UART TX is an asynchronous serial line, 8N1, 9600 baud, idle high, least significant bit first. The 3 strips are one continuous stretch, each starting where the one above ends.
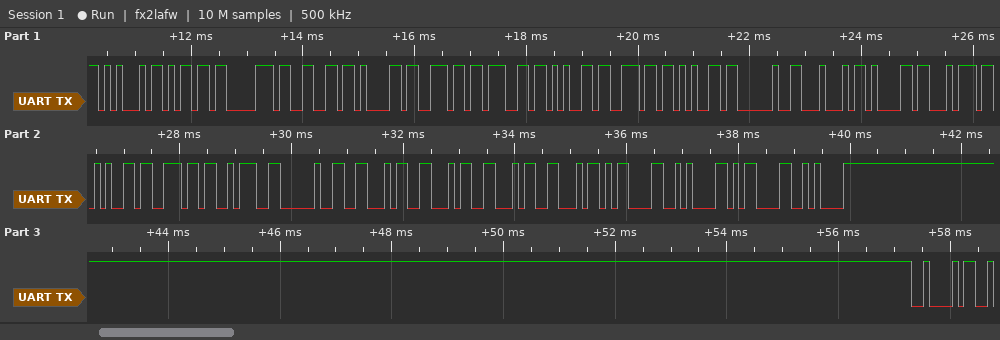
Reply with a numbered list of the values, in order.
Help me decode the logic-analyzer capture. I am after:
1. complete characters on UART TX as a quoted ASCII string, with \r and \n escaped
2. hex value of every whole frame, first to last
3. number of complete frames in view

1. "Empfangene Daten: FFFF\r\n\r\nB"
2. 0x45 0x6D 0x70 0x66 0x61 0x6E 0x67 0x65 0x6E 0x65 0x20 0x44 0x61 0x74 0x65 0x6E 0x3A 0x20 0x46 0x46 0x46 0x46 0x0D 0x0A 0x0D 0x0A 0x42
3. 27
